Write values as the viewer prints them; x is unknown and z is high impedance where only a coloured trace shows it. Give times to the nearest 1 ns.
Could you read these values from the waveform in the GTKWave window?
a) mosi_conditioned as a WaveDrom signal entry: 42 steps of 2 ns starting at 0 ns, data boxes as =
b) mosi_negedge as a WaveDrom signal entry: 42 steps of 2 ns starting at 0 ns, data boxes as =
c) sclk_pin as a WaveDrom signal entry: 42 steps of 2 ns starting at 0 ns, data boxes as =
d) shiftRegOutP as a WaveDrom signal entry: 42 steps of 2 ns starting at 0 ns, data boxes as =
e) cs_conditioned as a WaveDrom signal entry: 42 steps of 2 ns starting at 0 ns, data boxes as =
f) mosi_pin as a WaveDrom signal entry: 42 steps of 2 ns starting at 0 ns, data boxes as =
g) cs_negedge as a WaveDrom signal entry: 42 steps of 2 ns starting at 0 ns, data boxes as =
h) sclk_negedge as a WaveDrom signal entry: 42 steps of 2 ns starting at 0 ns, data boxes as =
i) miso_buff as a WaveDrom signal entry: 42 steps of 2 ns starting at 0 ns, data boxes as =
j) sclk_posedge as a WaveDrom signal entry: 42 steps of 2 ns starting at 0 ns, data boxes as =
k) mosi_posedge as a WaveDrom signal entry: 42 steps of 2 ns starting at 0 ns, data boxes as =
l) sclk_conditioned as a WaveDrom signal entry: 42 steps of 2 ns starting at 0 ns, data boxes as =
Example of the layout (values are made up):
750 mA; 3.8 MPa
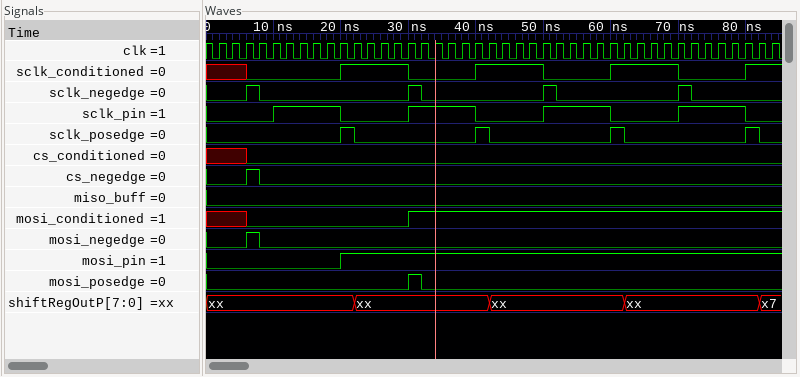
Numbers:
{name: 'mosi_conditioned', wave: 'x..0...........1..........................'}; {name: 'mosi_negedge', wave: '0..10.....................................'}; {name: 'sclk_pin', wave: '0....1....0....1....0....1....0....1....0.'}; {name: 'shiftRegOutP', wave: 'x..........=.........=.........=.........=', data: 'xx xx xx x7'}; {name: 'cs_conditioned', wave: 'x..0......................................'}; {name: 'mosi_pin', wave: '0.........1...............................'}; {name: 'cs_negedge', wave: '0..10.....................................'}; {name: 'sclk_negedge', wave: '0..10..........10........10........10.....'}; {name: 'miso_buff', wave: '0.........................................'}; {name: 'sclk_posedge', wave: '0.........10........10........10........10'}; {name: 'mosi_posedge', wave: '0..............10.........................'}; {name: 'sclk_conditioned', wave: 'x..0......1....0....1....0....1....0....1.'}
